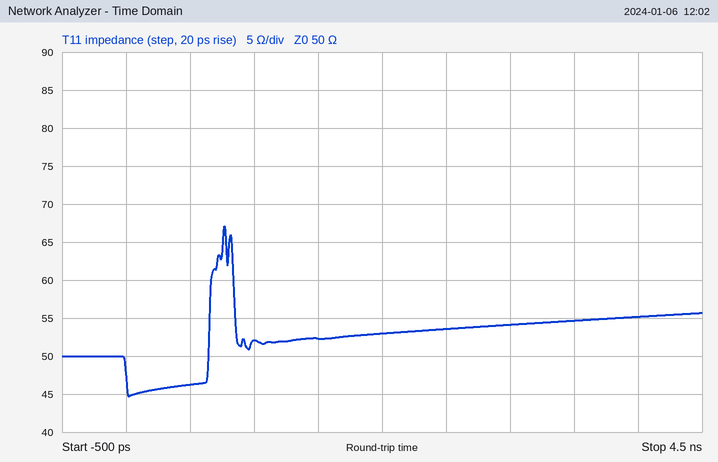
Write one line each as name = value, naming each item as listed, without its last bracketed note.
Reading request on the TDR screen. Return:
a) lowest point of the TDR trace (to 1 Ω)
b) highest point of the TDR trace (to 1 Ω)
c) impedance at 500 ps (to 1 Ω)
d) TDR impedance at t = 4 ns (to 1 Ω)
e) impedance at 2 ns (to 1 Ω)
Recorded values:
lowest point of the TDR trace = 45 Ω
highest point of the TDR trace = 67 Ω
impedance at 500 ps = 46 Ω
TDR impedance at t = 4 ns = 55 Ω
impedance at 2 ns = 53 Ω
